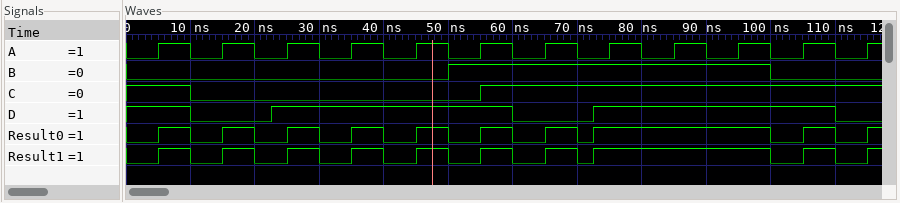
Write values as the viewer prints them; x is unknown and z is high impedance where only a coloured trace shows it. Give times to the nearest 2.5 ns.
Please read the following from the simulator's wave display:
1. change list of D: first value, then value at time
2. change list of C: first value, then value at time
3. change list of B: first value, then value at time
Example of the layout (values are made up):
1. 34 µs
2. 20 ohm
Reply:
1. 1, 0 at 10 ns, 1 at 22.5 ns, 0 at 60 ns, 1 at 72.5 ns, 0 at 110 ns
2. 1, 0 at 10 ns, 1 at 55 ns
3. 0, 1 at 50 ns, 0 at 100 ns
